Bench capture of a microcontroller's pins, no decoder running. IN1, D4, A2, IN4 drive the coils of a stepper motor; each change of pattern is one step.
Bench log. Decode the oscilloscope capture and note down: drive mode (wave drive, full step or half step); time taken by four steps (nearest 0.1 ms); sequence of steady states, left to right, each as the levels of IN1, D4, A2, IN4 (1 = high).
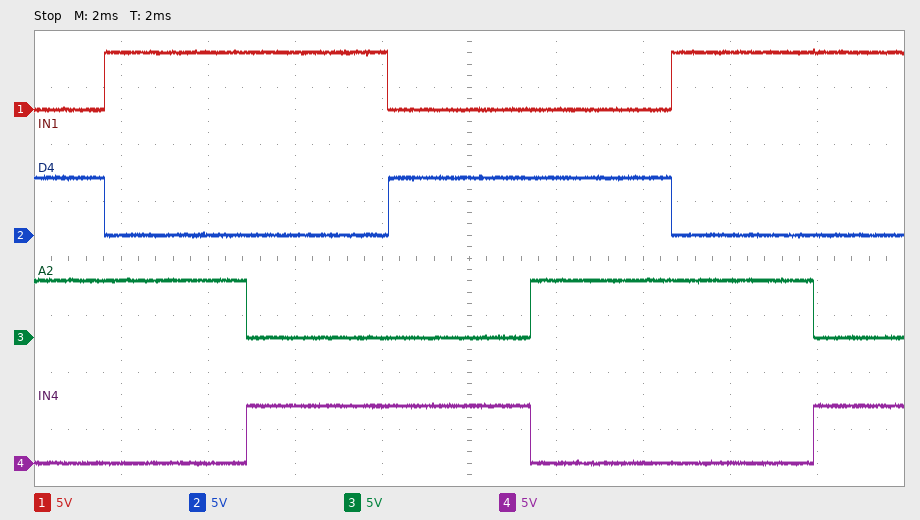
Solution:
full step
13.0 ms
0110 1010 1001 0101 0110 1010 1001
